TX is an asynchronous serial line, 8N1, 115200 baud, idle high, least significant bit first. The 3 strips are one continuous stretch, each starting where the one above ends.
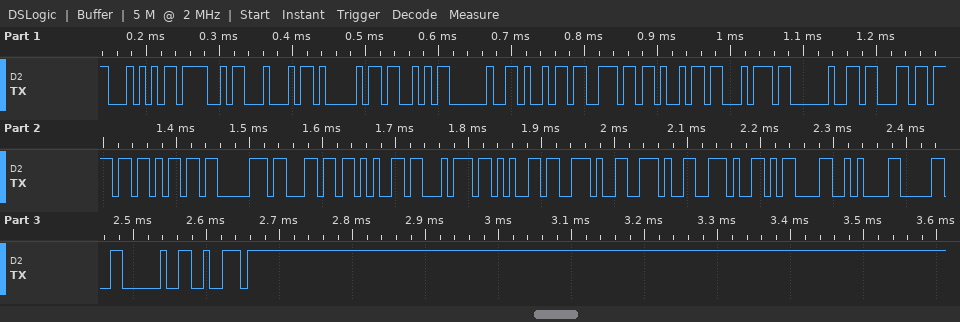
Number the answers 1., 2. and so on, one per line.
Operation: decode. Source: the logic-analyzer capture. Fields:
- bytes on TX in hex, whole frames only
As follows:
1. 0x54 0x4F 0x44 0x41 0x53 0x20 0x69 0x6E 0x69 0x74 0x20 0x63 0x6F 0x6D 0x70 0x6C 0x65 0x74 0x65 0x2E 0x2E 0x2E 0x0D 0x0A 0x30 0x20 0x72
